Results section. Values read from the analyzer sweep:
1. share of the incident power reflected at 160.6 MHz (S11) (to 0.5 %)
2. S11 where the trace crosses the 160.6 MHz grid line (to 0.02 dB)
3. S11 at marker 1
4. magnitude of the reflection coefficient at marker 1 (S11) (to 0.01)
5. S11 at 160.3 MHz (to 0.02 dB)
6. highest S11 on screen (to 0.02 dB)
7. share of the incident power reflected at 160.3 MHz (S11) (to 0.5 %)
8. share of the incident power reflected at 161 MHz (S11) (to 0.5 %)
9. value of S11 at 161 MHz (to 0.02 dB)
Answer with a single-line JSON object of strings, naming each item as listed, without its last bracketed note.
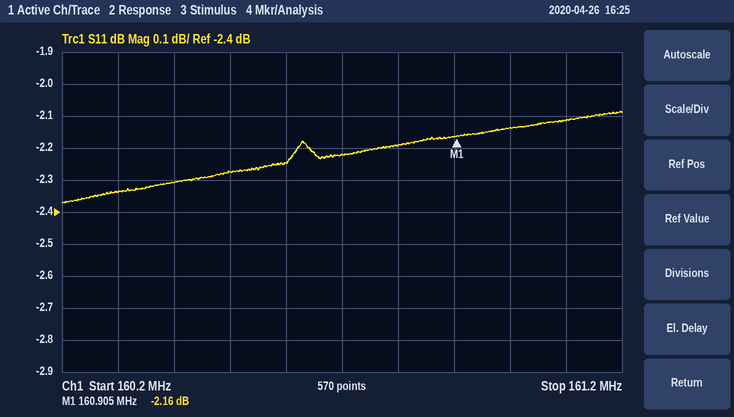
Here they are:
{"share of the incident power reflected at 160.6 MHz (S11)": "59.5 %", "S11 where the trace crosses the 160.6 MHz grid line": "-2.24 dB", "S11 at marker 1": "-2.16 dB", "magnitude of the reflection coefficient at marker 1 (S11)": "0.78", "S11 at 160.3 MHz": "-2.34 dB", "highest S11 on screen": "-2.08 dB", "share of the incident power reflected at 160.3 MHz (S11)": "58.5 %", "share of the incident power reflected at 161 MHz (S11)": "61.0 %", "value of S11 at 161 MHz": "-2.14 dB"}
